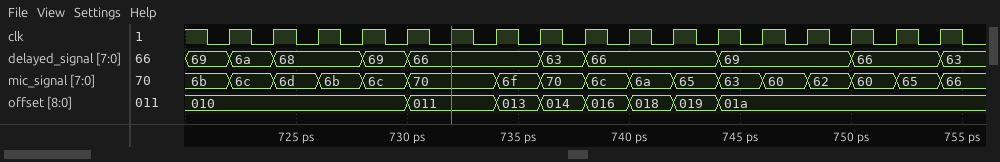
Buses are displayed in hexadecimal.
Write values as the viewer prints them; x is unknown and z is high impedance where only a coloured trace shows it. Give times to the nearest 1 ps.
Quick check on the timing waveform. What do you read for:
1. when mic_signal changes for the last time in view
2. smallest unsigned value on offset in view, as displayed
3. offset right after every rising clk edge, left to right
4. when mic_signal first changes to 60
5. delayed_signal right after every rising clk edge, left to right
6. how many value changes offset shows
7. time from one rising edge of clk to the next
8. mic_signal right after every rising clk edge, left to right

754 ps
010
010, 010, 010, 010, 011, 011, 013, 014, 016, 018, 019, 01a, 01a, 01a, 01a, 01a, 01a
746 ps
6a, 68, 68, 69, 66, 66, 66, 63, 66, 66, 66, 69, 69, 69, 66, 66, 63
7
2 ps
6c, 6d, 6b, 6c, 70, 70, 6f, 70, 6c, 6a, 65, 63, 60, 62, 60, 65, 66
